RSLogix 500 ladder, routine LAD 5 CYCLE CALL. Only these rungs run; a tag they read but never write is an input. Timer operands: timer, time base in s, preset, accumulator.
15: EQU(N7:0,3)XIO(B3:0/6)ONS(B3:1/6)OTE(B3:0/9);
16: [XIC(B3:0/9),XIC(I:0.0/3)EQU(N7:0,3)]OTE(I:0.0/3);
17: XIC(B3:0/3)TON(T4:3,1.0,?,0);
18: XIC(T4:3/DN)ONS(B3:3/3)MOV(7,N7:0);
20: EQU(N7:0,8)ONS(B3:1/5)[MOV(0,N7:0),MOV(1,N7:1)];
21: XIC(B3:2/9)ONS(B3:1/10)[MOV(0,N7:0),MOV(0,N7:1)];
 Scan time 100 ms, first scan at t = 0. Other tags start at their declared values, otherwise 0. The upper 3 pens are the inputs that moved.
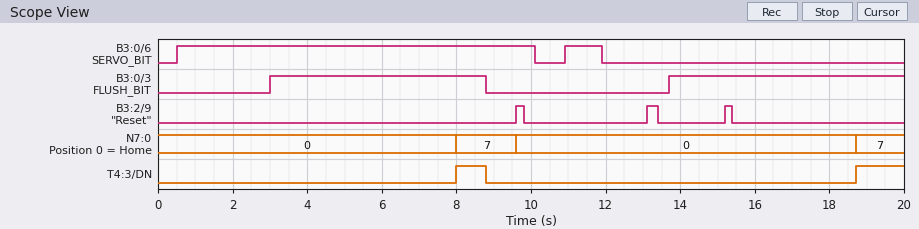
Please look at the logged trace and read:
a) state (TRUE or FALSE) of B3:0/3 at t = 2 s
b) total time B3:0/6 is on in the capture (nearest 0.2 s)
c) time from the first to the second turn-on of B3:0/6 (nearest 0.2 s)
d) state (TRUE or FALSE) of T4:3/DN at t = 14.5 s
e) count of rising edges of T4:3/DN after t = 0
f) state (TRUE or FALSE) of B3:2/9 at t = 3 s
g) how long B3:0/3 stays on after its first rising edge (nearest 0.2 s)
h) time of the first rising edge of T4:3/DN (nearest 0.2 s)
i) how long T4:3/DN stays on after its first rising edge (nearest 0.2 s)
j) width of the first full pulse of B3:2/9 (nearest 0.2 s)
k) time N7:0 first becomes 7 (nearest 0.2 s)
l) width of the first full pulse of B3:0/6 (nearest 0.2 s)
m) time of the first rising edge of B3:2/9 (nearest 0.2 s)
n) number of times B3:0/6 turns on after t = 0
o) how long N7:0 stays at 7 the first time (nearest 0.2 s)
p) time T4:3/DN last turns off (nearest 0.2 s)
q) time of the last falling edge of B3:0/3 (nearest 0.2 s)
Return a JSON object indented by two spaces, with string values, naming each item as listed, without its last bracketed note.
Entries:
{
  "state (TRUE or FALSE) of B3:0/3 at t = 2 s": "FALSE",
  "total time B3:0/6 is on in the capture": "10.6 s",
  "time from the first to the second turn-on of B3:0/6": "10.4 s",
  "state (TRUE or FALSE) of T4:3/DN at t = 14.5 s": "FALSE",
  "count of rising edges of T4:3/DN after t = 0": "2",
  "state (TRUE or FALSE) of B3:2/9 at t = 3 s": "FALSE",
  "how long B3:0/3 stays on after its first rising edge": "5.8 s",
  "time of the first rising edge of T4:3/DN": "8.0 s",
  "how long T4:3/DN stays on after its first rising edge": "0.8 s",
  "width of the first full pulse of B3:2/9": "0.2 s",
  "time N7:0 first becomes 7": "8.0 s",
  "width of the first full pulse of B3:0/6": "9.6 s",
  "time of the first rising edge of B3:2/9": "9.6 s",
  "number of times B3:0/6 turns on after t = 0": "2",
  "how long N7:0 stays at 7 the first time": "1.6 s",
  "time T4:3/DN last turns off": "8.8 s",
  "time of the last falling edge of B3:0/3": "8.8 s"
}
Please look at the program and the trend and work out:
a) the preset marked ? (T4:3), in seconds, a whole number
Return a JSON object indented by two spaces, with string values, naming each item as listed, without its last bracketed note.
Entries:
{
  "the preset marked ? (T4:3), in seconds, a whole number": "5 s"
}
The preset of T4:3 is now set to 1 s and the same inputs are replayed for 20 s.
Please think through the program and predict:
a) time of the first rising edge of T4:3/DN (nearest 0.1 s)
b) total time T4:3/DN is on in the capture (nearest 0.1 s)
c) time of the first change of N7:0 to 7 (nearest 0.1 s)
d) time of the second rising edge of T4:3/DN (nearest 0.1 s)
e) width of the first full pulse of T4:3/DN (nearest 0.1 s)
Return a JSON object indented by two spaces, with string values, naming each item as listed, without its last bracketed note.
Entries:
{
  "time of the first rising edge of T4:3/DN": "4.0 s",
  "total time T4:3/DN is on in the capture": "10.1 s",
  "time of the first change of N7:0 to 7": "4.0 s",
  "time of the second rising edge of T4:3/DN": "14.7 s",
  "width of the first full pulse of T4:3/DN": "4.8 s"
}
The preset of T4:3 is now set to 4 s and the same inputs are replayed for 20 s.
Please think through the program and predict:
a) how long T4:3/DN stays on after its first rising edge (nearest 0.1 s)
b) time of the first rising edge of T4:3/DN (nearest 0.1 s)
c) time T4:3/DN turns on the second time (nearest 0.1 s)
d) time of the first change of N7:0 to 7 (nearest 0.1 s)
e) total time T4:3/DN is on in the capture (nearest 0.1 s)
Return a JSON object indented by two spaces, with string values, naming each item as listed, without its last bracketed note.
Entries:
{
  "how long T4:3/DN stays on after its first rising edge": "1.8 s",
  "time of the first rising edge of T4:3/DN": "7.0 s",
  "time T4:3/DN turns on the second time": "17.7 s",
  "time of the first change of N7:0 to 7": "7.0 s",
  "total time T4:3/DN is on in the capture": "4.1 s"
}
